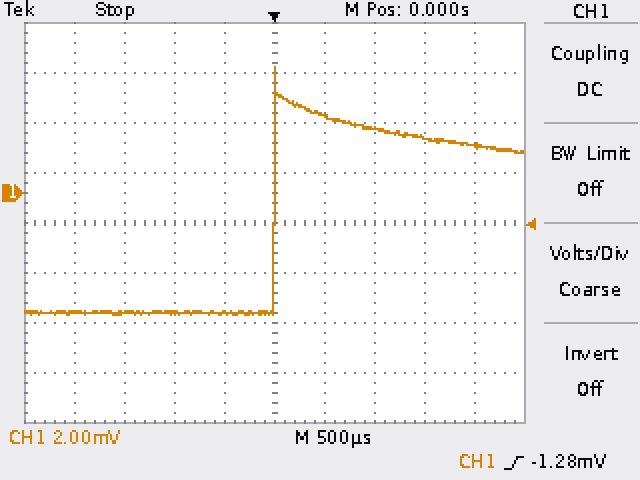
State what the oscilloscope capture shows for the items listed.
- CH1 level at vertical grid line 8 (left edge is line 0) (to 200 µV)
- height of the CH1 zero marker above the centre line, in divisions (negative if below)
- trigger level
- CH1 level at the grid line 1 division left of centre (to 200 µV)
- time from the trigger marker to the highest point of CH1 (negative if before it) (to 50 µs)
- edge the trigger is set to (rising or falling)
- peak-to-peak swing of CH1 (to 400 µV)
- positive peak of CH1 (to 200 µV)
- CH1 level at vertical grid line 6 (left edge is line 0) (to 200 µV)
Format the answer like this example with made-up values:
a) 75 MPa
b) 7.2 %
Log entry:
a) 2.2 mV
b) +0.6 div
c) -1.28 mV
d) -4.8 mV
e) 0 µs
f) rising
g) 10.0 mV
h) 5.0 mV
i) 3.0 mV
